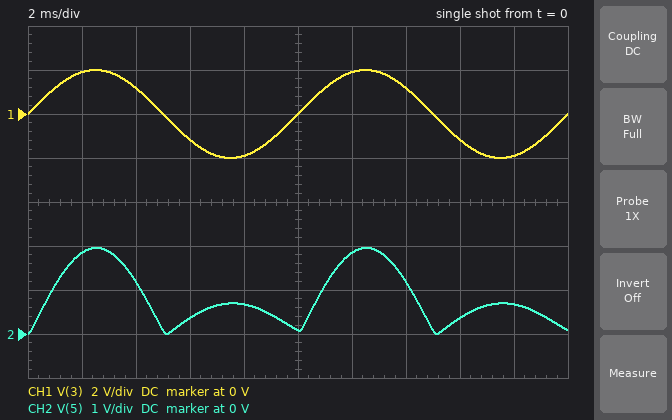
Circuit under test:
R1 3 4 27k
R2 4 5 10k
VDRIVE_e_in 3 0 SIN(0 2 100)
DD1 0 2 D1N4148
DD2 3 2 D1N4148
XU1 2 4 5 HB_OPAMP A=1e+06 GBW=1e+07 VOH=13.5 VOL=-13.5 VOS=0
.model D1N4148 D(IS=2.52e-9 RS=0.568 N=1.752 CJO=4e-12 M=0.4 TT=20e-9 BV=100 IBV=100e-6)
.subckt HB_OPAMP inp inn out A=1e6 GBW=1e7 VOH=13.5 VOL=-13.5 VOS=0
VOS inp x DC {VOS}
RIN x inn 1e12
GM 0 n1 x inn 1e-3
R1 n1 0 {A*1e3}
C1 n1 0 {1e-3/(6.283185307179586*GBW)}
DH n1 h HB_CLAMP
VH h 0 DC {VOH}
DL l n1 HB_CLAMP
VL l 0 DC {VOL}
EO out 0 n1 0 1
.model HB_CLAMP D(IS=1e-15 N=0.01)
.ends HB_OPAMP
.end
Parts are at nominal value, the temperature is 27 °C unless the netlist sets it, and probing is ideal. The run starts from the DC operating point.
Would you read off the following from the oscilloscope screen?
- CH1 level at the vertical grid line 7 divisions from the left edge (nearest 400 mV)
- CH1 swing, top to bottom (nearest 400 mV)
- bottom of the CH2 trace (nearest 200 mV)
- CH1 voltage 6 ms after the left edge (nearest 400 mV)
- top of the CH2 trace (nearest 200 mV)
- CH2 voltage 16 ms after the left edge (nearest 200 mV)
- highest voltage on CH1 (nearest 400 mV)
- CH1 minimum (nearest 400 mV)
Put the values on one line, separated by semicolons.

1.2 V; 4.0 V; 0 V; -1.2 V; 2.0 V; 400 mV; 2.0 V; -2.0 V
